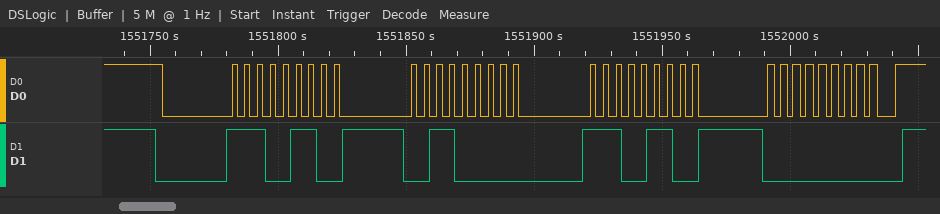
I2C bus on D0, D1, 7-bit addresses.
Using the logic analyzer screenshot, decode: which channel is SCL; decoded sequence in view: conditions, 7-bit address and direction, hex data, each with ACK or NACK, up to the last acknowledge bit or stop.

D0
start, address 73 write ACK, 30 ACK, E6 ACK, 00 ACK, stop
